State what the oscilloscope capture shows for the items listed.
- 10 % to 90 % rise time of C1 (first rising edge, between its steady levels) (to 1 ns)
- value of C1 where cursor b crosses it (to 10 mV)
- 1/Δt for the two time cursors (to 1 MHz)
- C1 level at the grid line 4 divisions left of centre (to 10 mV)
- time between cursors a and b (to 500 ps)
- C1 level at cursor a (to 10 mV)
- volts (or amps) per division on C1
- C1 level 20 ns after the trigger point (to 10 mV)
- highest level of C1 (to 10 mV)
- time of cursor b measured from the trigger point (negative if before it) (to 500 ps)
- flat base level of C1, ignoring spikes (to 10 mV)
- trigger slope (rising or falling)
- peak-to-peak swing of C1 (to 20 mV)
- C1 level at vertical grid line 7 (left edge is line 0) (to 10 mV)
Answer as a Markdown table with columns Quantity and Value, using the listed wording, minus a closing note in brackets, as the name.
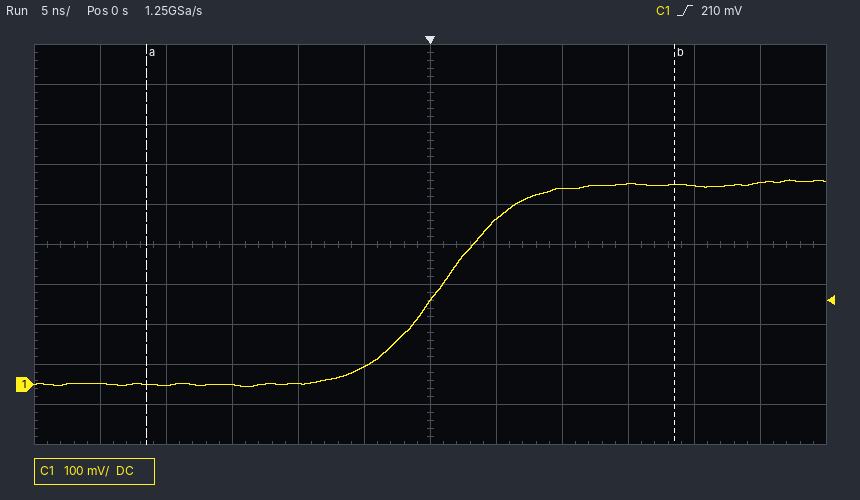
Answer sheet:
| Quantity | Value |
|---|---|
| 10 % to 90 % rise time of C1 (first rising edge, between its steady levels) | 11 ns |
| value of C1 where cursor b crosses it | 500 mV |
| 1/Δt for the two time cursors | 25 MHz |
| C1 level at the grid line 4 divisions left of centre | 0 mV |
| time between cursors a and b | 40.0 ns |
| C1 level at cursor a | 0 mV |
| volts (or amps) per division on C1 | 100 mV |
| C1 level 20 ns after the trigger point | 500 mV |
| highest level of C1 | 510 mV |
| time of cursor b measured from the trigger point (negative if before it) | +18.5 ns |
| flat base level of C1, ignoring spikes | 0 mV |
| trigger slope | rising |
| peak-to-peak swing of C1 | 520 mV |
| C1 level at vertical grid line 7 (left edge is line 0) | 410 mV |
